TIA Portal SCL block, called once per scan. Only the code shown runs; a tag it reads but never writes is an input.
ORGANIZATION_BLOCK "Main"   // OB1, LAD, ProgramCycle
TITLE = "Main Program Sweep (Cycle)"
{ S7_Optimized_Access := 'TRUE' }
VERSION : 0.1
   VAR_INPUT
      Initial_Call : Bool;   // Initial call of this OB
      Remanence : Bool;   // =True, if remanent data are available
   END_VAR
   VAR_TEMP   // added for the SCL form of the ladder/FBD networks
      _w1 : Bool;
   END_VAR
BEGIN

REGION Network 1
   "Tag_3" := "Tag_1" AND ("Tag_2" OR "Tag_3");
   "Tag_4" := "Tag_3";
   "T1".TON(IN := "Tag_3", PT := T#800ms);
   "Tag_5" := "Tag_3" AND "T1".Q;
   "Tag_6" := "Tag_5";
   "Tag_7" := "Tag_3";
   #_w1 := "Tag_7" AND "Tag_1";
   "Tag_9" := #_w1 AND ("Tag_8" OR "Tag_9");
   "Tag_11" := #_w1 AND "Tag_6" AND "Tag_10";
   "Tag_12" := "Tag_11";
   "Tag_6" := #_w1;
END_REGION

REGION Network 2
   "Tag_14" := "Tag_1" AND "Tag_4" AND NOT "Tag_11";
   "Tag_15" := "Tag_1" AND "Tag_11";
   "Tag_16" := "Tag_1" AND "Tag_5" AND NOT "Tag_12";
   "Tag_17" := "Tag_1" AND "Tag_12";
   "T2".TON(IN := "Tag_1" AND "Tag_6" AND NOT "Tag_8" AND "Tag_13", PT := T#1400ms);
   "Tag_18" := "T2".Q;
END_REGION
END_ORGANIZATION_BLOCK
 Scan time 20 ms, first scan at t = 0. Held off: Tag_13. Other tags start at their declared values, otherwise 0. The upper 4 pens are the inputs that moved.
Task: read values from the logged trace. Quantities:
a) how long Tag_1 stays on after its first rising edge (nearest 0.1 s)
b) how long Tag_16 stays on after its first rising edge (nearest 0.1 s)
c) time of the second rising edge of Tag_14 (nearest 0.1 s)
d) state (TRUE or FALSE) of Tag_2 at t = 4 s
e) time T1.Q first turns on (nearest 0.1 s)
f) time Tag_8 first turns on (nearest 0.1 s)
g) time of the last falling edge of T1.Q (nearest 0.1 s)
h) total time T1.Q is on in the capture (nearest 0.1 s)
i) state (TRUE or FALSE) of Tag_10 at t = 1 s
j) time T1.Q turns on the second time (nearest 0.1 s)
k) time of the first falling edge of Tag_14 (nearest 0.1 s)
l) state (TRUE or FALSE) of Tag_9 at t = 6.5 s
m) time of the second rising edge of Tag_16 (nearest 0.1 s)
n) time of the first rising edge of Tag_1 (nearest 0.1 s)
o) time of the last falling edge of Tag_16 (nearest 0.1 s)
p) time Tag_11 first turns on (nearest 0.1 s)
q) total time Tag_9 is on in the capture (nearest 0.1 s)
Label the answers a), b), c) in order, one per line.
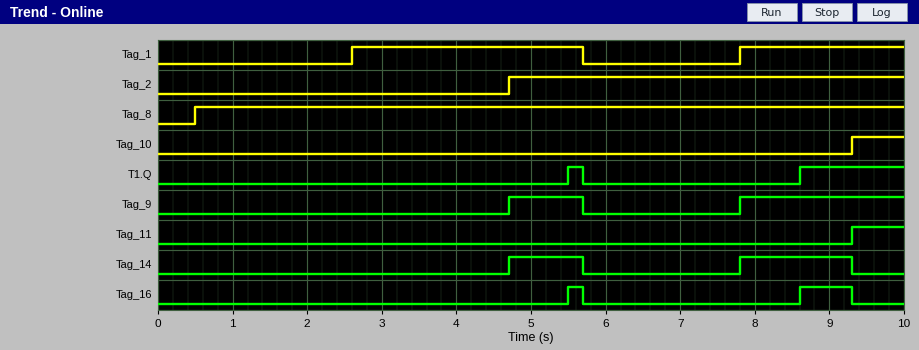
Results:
a) 3.1 s
b) 0.2 s
c) 7.8 s
d) FALSE
e) 5.5 s
f) 0.5 s
g) 5.7 s
h) 1.6 s
i) FALSE
j) 8.6 s
k) 5.7 s
l) FALSE
m) 8.6 s
n) 2.6 s
o) 9.3 s
p) 9.3 s
q) 3.2 s
